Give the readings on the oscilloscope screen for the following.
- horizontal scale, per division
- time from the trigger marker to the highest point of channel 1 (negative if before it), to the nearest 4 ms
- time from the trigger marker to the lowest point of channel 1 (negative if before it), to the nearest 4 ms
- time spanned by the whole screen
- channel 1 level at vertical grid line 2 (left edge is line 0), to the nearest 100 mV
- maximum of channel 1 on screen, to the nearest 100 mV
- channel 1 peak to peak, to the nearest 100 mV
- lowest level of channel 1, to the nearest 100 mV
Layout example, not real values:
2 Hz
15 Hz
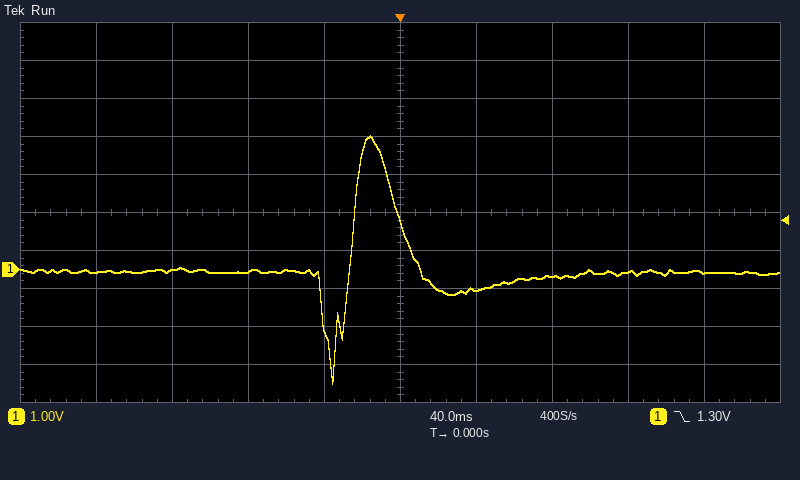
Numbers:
40 ms
-16 ms
-36 ms
400 ms
0.0 V
3.5 V
6.5 V
-3.0 V
